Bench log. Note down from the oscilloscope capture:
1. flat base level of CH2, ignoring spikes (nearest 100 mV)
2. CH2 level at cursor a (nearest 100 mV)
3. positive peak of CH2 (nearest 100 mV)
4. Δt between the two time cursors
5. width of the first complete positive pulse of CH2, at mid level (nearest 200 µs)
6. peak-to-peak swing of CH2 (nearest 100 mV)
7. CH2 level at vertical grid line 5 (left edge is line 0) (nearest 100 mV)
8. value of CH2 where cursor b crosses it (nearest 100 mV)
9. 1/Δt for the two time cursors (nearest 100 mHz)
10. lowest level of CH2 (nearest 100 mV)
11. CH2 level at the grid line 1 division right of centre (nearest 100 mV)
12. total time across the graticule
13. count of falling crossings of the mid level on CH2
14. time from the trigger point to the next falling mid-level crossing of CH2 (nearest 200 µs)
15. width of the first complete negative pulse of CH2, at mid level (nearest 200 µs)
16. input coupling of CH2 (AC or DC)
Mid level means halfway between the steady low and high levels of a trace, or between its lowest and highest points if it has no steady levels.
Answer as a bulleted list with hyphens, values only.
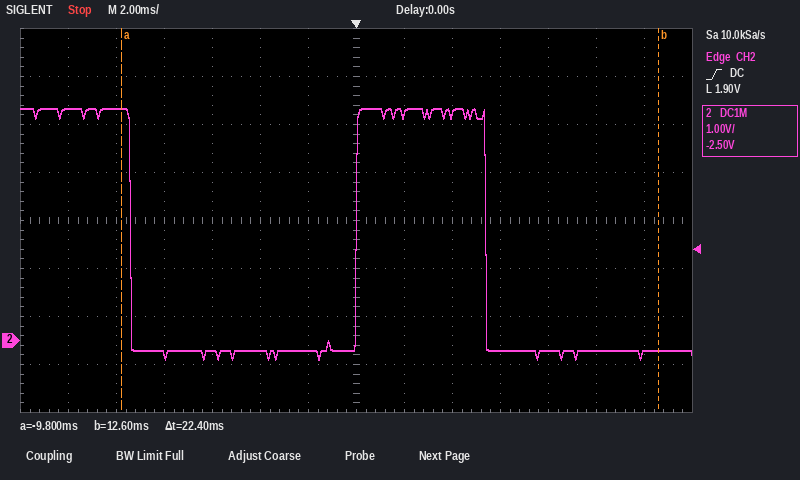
- -200 mV
- 4.8 V
- 4.8 V
- 22.4 ms
- 5.4 ms
- 5.2 V
- -200 mV
- -200 mV
- 44.6 Hz
- -400 mV
- 4.7 V
- 28 ms
- 2
- 5.4 ms
- 9.4 ms
- DC
